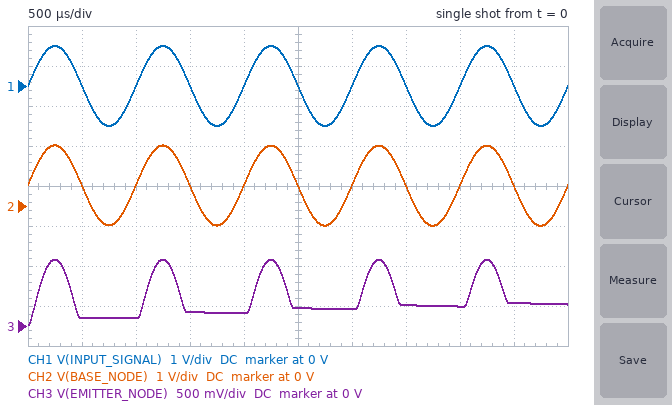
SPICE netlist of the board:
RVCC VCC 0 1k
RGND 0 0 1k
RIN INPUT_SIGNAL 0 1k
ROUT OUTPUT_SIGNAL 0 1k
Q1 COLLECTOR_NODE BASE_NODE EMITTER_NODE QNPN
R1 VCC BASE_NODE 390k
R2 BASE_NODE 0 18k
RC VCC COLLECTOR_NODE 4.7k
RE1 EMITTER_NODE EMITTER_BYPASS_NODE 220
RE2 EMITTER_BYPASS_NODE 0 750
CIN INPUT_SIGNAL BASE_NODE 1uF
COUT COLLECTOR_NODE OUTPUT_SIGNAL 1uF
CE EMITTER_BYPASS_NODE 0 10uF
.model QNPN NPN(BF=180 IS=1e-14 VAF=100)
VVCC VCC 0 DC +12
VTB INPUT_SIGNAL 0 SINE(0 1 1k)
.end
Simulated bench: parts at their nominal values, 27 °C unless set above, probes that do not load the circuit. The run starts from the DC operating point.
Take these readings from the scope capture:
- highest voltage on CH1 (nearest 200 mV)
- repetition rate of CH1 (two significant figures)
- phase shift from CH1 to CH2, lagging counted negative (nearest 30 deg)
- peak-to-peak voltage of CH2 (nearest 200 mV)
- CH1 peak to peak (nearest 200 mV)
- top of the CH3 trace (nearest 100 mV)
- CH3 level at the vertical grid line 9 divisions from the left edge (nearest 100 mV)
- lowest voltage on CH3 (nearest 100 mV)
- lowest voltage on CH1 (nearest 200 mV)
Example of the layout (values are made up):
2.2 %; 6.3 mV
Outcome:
1.0 V; 1.0 kHz; 0 deg; 2.0 V; 2.0 V; 800 mV; 300 mV; 0 V; -1.0 V
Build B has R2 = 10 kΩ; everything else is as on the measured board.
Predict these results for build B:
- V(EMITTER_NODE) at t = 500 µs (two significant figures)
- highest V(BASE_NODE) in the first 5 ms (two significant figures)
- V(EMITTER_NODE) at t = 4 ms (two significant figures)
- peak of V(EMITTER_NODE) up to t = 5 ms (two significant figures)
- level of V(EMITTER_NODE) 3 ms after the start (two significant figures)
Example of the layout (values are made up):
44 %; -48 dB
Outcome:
62 mV; 1.3 V; 160 mV; 610 mV; 130 mV
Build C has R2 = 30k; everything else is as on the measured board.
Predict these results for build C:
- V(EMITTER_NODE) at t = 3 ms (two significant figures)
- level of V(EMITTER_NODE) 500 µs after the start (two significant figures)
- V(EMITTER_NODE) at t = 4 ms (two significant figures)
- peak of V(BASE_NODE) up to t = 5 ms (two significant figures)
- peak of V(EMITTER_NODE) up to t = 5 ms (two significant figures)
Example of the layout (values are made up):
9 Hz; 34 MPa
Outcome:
370 mV; 280 mV; 410 mV; 1.8 V; 1.1 V
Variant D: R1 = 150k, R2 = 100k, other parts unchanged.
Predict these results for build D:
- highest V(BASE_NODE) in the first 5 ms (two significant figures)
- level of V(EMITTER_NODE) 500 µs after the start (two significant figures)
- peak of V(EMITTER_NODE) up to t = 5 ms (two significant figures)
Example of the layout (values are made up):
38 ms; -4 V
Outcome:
3.3 V; 1.6 V; 2.6 V
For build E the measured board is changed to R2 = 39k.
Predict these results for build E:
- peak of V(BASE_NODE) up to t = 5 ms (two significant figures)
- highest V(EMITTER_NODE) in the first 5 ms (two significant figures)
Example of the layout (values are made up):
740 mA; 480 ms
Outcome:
2.0 V; 1.3 V
